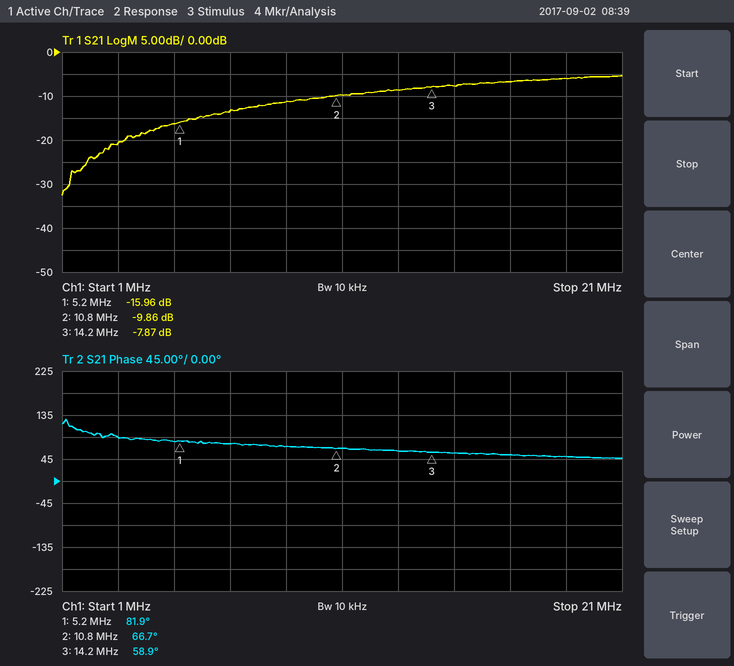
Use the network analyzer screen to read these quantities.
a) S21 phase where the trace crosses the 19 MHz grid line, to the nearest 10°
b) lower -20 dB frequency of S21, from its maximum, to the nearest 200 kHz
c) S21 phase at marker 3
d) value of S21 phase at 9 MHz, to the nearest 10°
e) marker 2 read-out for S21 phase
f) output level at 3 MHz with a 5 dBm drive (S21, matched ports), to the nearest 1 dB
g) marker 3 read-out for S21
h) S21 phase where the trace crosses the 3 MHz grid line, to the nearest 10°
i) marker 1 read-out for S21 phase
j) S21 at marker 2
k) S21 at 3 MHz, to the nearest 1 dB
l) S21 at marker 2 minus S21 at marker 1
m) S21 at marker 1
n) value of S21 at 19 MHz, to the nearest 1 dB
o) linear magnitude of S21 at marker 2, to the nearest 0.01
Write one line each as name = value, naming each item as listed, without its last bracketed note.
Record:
S21 phase where the trace crosses the 19 MHz grid line, to the nearest 10° = 50°
lower -20 dB frequency of S21, from its maximum, to the nearest 200 kHz = 1.8 MHz
S21 phase at marker 3 = 58.9°
value of S21 phase at 9 MHz, to the nearest 10° = 70°
marker 2 read-out for S21 phase = 66.7°
output level at 3 MHz with a 5 dBm drive (S21, matched ports), to the nearest 1 dB = -16 dBm
marker 3 read-out for S21 = -7.87 dB
S21 phase where the trace crosses the 3 MHz grid line, to the nearest 10° = 90°
marker 1 read-out for S21 phase = 81.9°
S21 at marker 2 = -9.86 dB
S21 at 3 MHz, to the nearest 1 dB = -21 dB
S21 at marker 2 minus S21 at marker 1 = 6.10 dB
S21 at marker 1 = -15.96 dB
value of S21 at 19 MHz, to the nearest 1 dB = -6 dB
linear magnitude of S21 at marker 2, to the nearest 0.01 = 0.32
